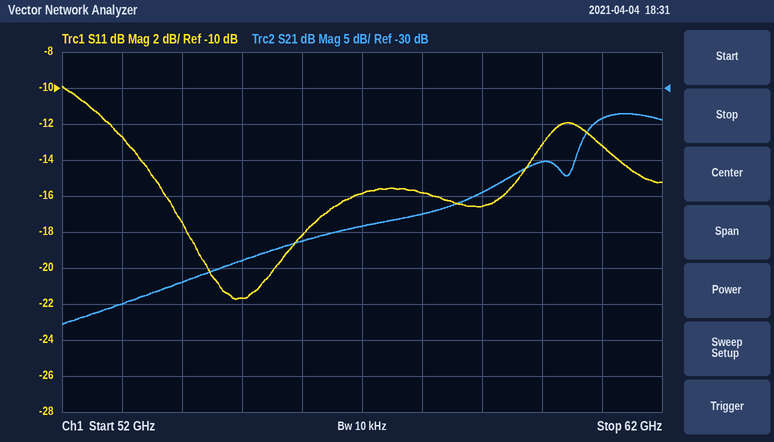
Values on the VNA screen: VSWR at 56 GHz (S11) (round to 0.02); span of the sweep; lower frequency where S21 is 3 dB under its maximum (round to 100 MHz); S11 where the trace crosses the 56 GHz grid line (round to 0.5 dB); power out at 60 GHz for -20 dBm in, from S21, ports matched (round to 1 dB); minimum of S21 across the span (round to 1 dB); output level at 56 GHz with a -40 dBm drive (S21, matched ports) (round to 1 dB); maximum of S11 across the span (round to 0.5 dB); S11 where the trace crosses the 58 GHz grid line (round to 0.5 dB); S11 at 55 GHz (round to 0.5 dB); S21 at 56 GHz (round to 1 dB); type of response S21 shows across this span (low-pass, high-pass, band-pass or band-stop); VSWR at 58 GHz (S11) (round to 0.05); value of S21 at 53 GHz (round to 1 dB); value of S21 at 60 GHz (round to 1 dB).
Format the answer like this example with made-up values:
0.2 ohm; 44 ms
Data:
1.28; 10 GHz; 60.7 GHz; -18.0 dB; -60 dBm; -63 dB; -91 dBm; -10.0 dB; -16.0 dB; -21.5 dB; -51 dB; high-pass; 1.40; -60 dB; -40 dB
